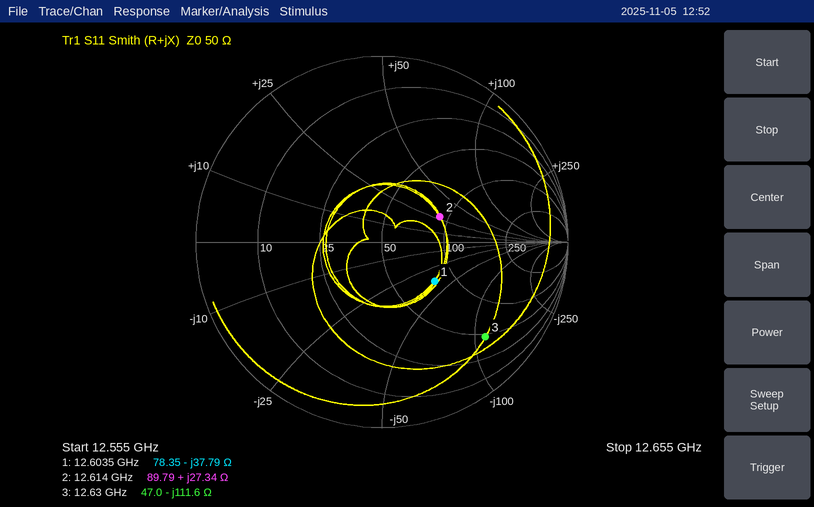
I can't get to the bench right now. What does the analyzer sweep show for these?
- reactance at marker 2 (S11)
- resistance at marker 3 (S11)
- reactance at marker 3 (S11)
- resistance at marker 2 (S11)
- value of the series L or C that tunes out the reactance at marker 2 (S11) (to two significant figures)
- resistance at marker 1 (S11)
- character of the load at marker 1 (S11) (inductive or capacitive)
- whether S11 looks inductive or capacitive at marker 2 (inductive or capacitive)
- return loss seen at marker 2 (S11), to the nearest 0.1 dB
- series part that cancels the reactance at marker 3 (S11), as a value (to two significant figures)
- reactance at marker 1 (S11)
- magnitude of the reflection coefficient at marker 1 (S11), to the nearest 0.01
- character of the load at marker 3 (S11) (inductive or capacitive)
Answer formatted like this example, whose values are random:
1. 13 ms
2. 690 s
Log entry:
1. +27.34 Ω
2. 47.0 Ω
3. -111.6 Ω
4. 89.79 Ω
5. 460 fF
6. 78.35 Ω
7. capacitive
8. inductive
9. 9.4 dB
10. 1.4 nH
11. -37.79 Ω
12. 0.35
13. capacitive
